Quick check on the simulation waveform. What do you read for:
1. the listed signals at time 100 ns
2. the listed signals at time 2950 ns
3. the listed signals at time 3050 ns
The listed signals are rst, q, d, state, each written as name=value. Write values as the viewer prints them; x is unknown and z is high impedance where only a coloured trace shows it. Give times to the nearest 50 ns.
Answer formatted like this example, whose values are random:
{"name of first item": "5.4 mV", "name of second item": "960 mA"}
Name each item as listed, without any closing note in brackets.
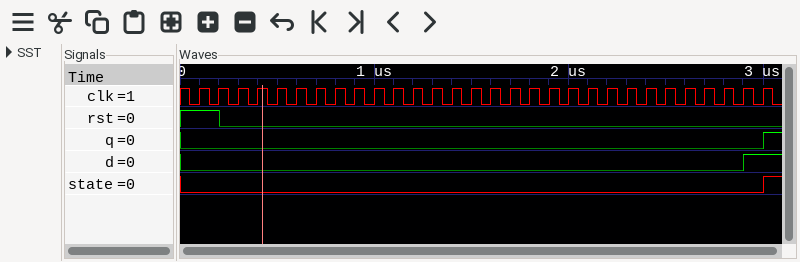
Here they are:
{"the listed signals at time 100 ns": "rst=1, q=0, d=0, state=0", "the listed signals at time 2950 ns": "rst=0, q=0, d=1, state=0", "the listed signals at time 3050 ns": "rst=0, q=1, d=1, state=1"}
